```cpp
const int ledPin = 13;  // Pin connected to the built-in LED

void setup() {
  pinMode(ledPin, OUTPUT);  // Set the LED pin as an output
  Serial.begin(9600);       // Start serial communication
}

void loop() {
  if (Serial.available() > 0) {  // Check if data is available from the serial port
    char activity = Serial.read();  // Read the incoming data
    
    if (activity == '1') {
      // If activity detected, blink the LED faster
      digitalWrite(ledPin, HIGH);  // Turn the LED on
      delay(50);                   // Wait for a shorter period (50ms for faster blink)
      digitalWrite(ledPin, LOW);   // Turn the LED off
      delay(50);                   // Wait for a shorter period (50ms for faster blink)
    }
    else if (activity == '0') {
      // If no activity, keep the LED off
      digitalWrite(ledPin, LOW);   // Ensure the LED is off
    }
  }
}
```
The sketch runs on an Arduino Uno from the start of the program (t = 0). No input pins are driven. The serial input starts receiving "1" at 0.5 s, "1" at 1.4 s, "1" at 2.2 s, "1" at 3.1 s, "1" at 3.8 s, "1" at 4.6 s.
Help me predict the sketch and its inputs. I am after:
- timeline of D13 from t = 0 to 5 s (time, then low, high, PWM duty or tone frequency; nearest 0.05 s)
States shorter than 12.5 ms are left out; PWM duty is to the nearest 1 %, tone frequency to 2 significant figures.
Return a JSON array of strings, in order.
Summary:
["0 s low; 0.5 s high; 0.55 s low; 1.4 s high; 1.45 s low; 2.2 s high; 2.25 s low; 3.1 s high; 3.15 s low; 3.8 s high; 3.85 s low; 4.6 s high; 4.65 s low"]
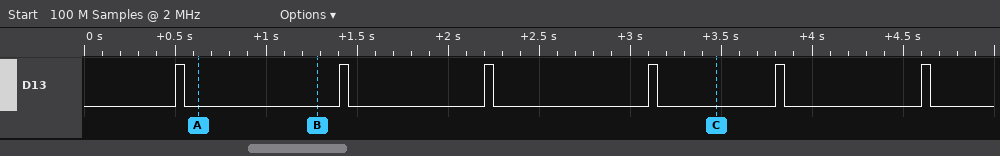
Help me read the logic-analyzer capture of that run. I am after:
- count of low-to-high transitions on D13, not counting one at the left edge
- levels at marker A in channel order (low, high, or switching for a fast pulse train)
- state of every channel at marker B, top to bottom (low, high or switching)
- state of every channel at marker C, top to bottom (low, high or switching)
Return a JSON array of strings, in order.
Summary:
["6", "D13 low", "D13 low", "D13 low"]
